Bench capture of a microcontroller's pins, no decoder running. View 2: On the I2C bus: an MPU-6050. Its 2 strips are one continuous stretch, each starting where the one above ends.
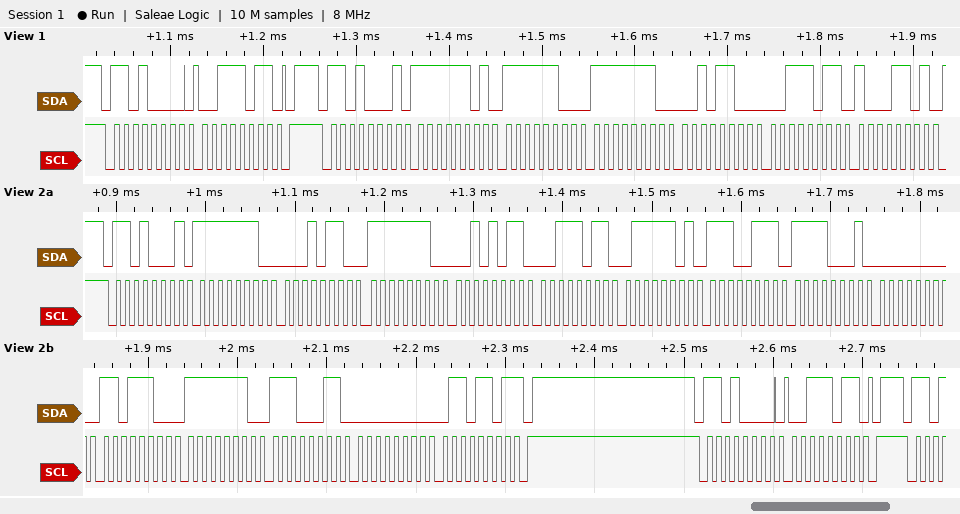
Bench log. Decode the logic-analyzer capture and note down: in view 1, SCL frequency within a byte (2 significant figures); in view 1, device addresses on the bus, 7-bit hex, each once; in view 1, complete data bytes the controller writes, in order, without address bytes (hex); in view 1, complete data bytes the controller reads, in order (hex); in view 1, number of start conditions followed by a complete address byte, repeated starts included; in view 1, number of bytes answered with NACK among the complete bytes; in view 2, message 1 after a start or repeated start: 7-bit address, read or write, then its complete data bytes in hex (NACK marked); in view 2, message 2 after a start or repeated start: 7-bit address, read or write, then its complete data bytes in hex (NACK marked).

100 kHz
0x68
3B
FD FC FE 2C 3B 8D
2
0
0x68 read: FE 16 FE 2B 3B 7D E7 F1 00 DC FE E3 00 6D NACK
0x68 write: 3B
